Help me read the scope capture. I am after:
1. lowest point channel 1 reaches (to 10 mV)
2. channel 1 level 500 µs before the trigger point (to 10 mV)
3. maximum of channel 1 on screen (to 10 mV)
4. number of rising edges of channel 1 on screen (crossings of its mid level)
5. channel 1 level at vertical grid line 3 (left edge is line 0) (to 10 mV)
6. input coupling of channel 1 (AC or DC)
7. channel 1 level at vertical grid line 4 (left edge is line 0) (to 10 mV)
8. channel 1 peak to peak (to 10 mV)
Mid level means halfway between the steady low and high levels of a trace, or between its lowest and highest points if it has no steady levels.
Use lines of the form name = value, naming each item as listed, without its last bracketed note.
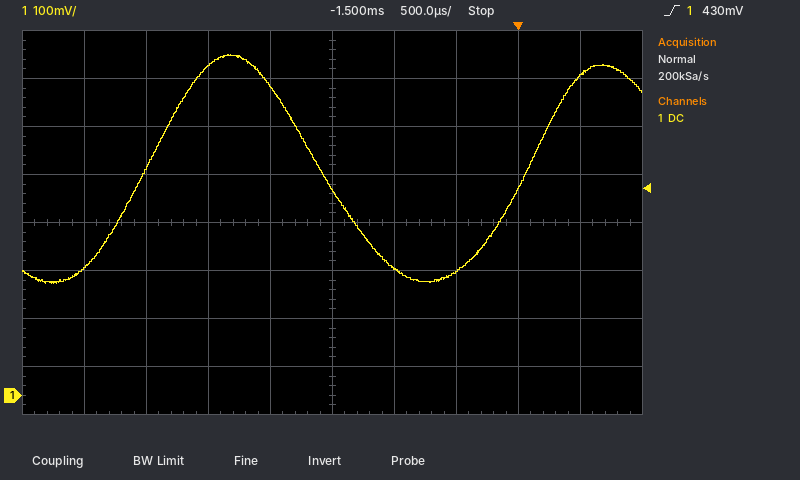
lowest point channel 1 reaches = 230 mV
channel 1 level 500 µs before the trigger point = 260 mV
maximum of channel 1 on screen = 710 mV
number of rising edges of channel 1 on screen = 2
channel 1 level at vertical grid line 3 (left edge is line 0) = 690 mV
input coupling of channel 1 = DC
channel 1 level at vertical grid line 4 (left edge is line 0) = 640 mV
channel 1 peak to peak = 480 mV
